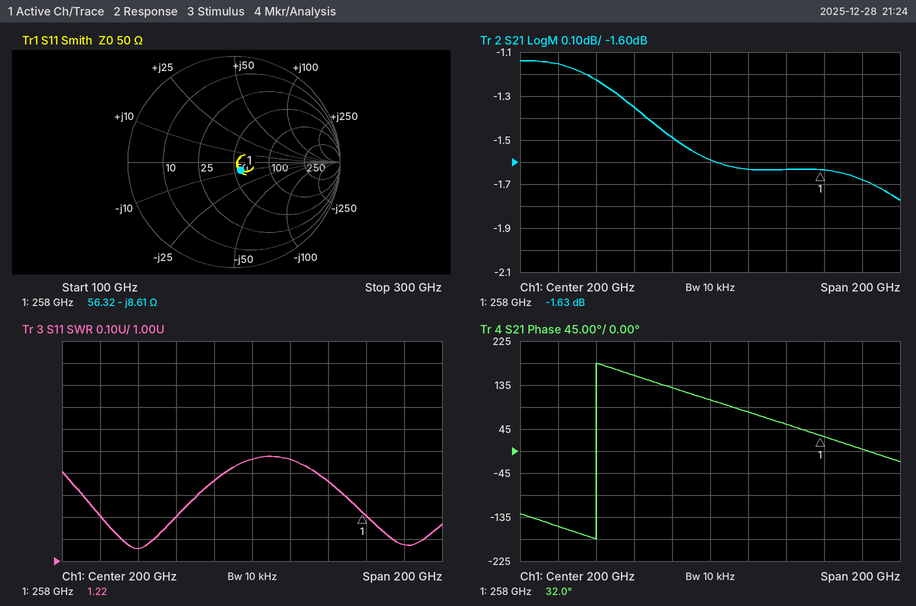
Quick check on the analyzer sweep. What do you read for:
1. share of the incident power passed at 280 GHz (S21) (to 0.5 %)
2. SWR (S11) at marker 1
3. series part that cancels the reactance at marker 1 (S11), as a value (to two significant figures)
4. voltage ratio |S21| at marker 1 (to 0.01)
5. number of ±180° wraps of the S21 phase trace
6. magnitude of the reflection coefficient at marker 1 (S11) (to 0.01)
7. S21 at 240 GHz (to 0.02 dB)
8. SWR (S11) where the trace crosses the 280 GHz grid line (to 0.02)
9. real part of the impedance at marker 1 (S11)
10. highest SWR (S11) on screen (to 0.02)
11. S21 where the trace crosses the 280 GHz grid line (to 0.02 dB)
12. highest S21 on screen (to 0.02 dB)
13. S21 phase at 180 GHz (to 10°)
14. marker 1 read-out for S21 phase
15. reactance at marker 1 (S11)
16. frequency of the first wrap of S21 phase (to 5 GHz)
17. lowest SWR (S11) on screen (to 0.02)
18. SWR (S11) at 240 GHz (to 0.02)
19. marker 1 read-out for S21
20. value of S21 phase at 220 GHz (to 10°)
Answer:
68.0 %
1.22
5.3 pH
0.83
1
0.10
-1.64 dB
1.08
56.32 Ω
1.48
-1.68 dB
-1.14 dB
130°
32.0°
-8.61 Ω
140 GHz
1.06
1.36
-1.63 dB
80°
